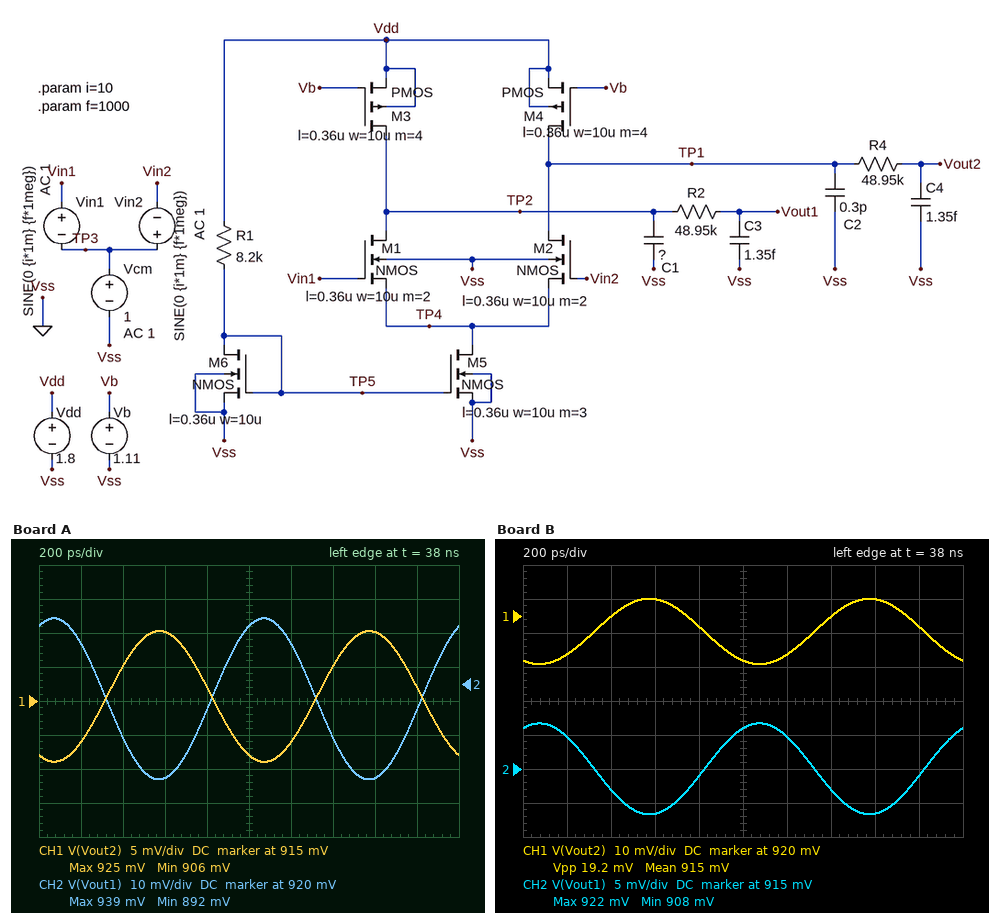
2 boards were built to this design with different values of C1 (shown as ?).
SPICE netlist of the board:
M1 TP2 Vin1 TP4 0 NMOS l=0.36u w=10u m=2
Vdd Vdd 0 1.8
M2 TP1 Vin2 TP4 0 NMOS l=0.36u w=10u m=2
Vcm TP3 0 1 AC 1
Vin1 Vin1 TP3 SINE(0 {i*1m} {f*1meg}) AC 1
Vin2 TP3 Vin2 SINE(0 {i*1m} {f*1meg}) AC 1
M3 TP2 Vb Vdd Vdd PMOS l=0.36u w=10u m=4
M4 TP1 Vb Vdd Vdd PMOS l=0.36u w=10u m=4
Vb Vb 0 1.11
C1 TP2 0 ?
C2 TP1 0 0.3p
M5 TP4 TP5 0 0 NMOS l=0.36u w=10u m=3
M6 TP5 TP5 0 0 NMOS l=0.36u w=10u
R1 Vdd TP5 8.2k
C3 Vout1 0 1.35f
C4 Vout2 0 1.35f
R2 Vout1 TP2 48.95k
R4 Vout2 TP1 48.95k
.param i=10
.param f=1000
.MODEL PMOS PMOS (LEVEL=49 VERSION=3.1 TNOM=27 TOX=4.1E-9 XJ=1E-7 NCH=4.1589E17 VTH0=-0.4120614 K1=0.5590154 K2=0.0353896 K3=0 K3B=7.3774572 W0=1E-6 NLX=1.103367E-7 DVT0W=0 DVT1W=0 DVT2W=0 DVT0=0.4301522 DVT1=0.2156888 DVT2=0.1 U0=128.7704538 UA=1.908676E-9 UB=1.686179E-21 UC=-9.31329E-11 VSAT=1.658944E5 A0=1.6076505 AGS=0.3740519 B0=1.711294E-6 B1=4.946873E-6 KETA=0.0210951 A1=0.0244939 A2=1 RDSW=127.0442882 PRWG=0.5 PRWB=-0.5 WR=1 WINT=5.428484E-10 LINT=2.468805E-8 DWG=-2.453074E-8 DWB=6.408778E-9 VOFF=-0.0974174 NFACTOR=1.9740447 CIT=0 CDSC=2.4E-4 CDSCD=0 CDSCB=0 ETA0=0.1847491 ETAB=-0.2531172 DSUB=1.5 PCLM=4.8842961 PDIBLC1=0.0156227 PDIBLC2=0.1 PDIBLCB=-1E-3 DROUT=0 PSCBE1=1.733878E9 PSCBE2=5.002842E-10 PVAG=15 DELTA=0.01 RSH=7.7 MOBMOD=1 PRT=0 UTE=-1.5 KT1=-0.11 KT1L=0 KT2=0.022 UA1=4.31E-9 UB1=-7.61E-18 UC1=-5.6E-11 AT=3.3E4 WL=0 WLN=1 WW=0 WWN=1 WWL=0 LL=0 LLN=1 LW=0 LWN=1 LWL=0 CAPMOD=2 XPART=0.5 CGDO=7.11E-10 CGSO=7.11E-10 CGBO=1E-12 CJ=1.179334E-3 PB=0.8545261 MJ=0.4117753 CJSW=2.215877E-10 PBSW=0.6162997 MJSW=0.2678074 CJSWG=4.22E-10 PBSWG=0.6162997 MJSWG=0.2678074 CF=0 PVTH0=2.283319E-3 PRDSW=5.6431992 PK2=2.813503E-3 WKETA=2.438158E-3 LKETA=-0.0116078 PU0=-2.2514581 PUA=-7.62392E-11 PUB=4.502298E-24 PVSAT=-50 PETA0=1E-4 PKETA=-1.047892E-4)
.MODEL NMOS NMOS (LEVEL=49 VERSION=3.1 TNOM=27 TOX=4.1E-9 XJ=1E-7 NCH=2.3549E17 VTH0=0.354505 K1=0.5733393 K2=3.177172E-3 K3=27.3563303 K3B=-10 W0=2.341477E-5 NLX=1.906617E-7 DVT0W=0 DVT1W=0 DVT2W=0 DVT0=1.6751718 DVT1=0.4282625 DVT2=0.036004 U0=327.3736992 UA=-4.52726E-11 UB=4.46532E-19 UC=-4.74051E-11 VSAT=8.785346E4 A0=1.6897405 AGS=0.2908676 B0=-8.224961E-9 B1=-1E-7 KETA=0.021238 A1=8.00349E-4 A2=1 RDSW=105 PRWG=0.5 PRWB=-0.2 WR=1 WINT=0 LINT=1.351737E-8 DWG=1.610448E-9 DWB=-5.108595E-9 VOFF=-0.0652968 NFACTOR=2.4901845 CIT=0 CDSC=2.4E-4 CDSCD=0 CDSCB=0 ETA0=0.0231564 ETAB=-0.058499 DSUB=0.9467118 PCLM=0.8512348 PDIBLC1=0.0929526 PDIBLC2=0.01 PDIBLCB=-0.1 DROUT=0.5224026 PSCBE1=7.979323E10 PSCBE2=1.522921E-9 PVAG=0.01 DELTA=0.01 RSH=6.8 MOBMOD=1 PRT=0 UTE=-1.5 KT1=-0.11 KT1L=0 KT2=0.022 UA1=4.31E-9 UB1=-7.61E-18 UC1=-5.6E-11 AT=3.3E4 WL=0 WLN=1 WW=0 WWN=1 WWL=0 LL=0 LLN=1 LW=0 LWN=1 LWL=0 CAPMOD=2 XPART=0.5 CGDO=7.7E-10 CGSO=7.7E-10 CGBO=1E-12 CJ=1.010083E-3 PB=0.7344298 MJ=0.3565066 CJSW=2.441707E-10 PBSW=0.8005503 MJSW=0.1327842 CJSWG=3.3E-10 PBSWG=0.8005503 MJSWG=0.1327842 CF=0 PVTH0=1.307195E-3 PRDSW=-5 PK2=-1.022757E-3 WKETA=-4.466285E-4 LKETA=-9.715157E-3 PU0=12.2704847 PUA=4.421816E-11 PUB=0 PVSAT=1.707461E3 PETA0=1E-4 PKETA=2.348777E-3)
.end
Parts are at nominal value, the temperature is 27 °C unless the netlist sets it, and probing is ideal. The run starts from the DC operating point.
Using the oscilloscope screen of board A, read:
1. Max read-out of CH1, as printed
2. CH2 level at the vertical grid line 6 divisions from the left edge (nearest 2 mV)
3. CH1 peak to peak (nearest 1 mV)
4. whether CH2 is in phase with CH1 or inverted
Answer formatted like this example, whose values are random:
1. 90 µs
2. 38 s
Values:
1. 925 mV
2. 932 mV
3. 19 mV
4. inverted
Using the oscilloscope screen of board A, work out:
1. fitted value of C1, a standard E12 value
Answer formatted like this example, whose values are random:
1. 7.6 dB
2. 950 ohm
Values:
1. 100 fF
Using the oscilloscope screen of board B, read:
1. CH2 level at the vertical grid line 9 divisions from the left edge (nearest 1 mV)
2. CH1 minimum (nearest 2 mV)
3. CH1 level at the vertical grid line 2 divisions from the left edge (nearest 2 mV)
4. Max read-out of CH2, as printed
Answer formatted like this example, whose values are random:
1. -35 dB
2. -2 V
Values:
1. 914 mV
2. 906 mV
3. 920 mV
4. 922 mV
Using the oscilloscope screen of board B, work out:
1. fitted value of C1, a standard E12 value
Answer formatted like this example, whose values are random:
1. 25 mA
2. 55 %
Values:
1. 470 fF
